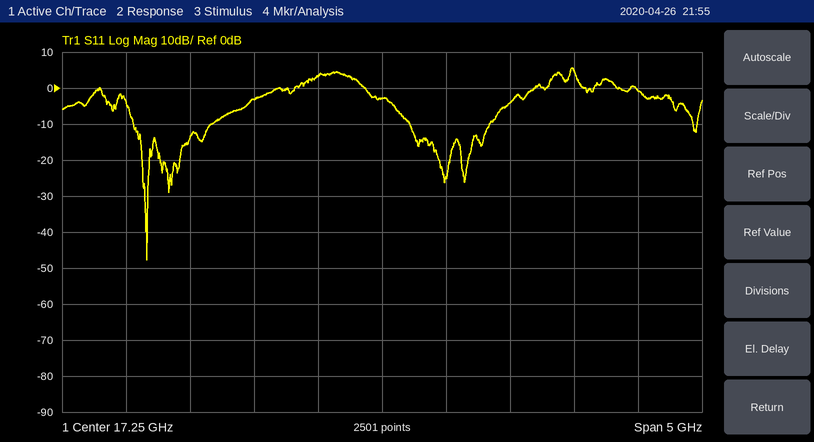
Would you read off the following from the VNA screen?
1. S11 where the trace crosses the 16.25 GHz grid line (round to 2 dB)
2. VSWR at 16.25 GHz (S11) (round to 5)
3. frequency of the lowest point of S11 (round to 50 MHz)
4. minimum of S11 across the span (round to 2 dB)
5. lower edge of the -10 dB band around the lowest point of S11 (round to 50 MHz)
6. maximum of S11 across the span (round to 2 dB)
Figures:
-4 dB
5
15.40 GHz
-48 dB
15.30 GHz
6 dB
